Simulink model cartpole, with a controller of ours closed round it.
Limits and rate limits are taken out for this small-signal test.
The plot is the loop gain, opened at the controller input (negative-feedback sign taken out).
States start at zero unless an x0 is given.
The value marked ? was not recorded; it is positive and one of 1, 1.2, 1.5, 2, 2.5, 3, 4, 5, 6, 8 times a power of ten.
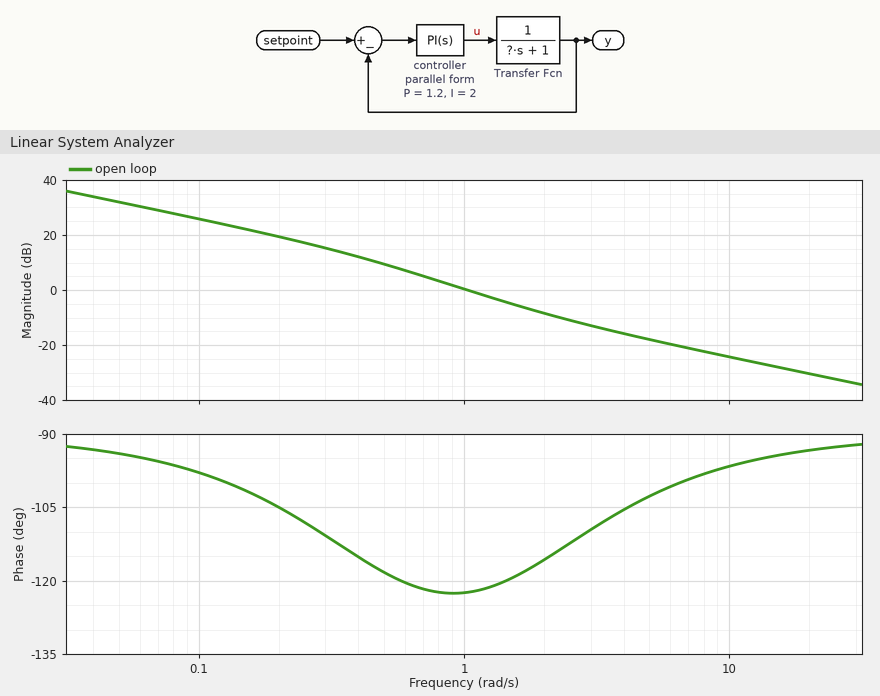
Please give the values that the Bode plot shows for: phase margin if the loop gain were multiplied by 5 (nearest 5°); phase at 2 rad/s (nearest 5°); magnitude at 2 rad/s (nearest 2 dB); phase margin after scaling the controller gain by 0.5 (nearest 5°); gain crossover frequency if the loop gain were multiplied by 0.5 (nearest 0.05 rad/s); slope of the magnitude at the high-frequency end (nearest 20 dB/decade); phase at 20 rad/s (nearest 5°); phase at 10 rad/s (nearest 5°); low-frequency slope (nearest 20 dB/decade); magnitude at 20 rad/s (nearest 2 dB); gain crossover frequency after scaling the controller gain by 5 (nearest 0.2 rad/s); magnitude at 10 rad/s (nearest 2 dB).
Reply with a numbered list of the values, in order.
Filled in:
1. 70°
2. -115°
3. -8 dB
4. 60°
5. 0.65 rad/s
6. -20 dB/decade
7. -95°
8. -95°
9. -20 dB/decade
10. -30 dB
11. 3.4 rad/s
12. -24 dB
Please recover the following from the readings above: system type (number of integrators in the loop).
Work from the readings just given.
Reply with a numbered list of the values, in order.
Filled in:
1. 1
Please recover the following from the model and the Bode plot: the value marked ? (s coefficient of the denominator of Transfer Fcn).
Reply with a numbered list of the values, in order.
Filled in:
1. 2
